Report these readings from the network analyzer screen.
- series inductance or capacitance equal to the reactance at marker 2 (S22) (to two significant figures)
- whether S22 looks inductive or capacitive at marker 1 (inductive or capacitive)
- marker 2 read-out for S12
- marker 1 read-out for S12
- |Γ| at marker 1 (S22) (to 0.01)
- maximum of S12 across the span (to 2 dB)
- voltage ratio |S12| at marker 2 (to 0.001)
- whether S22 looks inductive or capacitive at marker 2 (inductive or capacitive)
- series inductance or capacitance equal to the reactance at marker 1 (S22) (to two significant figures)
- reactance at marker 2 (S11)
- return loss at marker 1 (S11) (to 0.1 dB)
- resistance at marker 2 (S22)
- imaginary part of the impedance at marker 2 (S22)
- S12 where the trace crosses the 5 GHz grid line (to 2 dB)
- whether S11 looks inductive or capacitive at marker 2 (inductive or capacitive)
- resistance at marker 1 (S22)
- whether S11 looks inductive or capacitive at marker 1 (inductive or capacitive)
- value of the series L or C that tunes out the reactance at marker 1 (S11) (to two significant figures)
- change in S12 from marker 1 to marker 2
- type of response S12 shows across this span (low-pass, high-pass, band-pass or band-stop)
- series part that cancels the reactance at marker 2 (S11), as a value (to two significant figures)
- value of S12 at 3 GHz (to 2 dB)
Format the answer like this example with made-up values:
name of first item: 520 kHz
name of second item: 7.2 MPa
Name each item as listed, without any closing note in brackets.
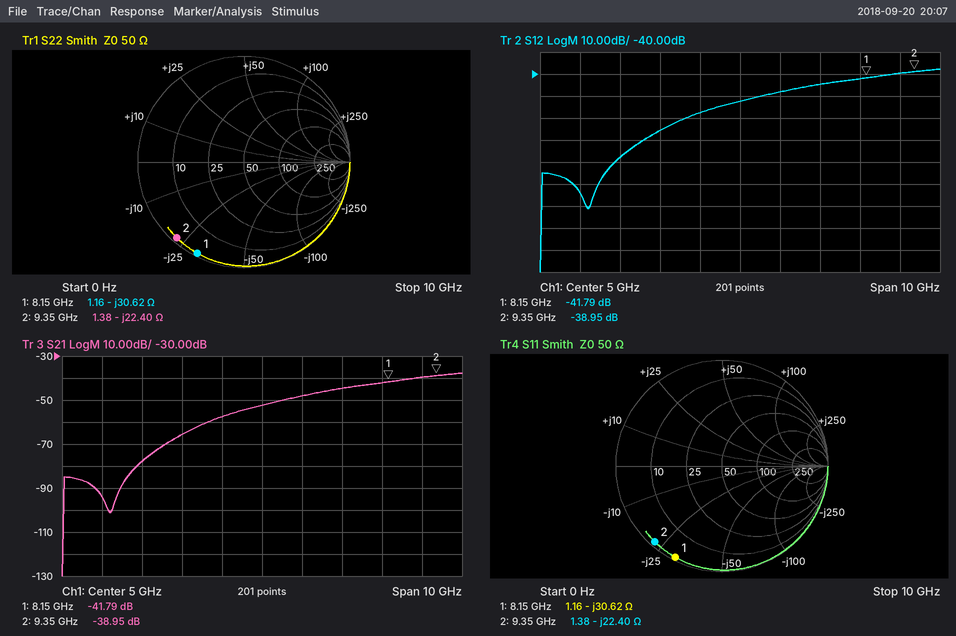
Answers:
series inductance or capacitance equal to the reactance at marker 2 (S22): 760 fF
whether S22 looks inductive or capacitive at marker 1: capacitive
marker 2 read-out for S12: -38.95 dB
marker 1 read-out for S12: -41.79 dB
|Γ| at marker 1 (S22): 0.97
maximum of S12 across the span: -38 dB
voltage ratio |S12| at marker 2: 0.011
whether S22 looks inductive or capacitive at marker 2: capacitive
series inductance or capacitance equal to the reactance at marker 1 (S22): 640 fF
reactance at marker 2: -22.40 Ω
return loss at marker 1 (S11): 0.3 dB
resistance at marker 2: 1.38 Ω
imaginary part of the impedance at marker 2: -22.40 Ω
S12 where the trace crosses the 5 GHz grid line: -52 dB
whether S11 looks inductive or capacitive at marker 2: capacitive
resistance at marker 1: 1.16 Ω
whether S11 looks inductive or capacitive at marker 1: capacitive
value of the series L or C that tunes out the reactance at marker 1 (S11): 600 pH
change in S12 from marker 1 to marker 2: 2.84 dB
type of response S12 shows across this span: high-pass
series part that cancels the reactance at marker 2 (S11), as a value: 380 pH
value of S12 at 3 GHz: -66 dB
